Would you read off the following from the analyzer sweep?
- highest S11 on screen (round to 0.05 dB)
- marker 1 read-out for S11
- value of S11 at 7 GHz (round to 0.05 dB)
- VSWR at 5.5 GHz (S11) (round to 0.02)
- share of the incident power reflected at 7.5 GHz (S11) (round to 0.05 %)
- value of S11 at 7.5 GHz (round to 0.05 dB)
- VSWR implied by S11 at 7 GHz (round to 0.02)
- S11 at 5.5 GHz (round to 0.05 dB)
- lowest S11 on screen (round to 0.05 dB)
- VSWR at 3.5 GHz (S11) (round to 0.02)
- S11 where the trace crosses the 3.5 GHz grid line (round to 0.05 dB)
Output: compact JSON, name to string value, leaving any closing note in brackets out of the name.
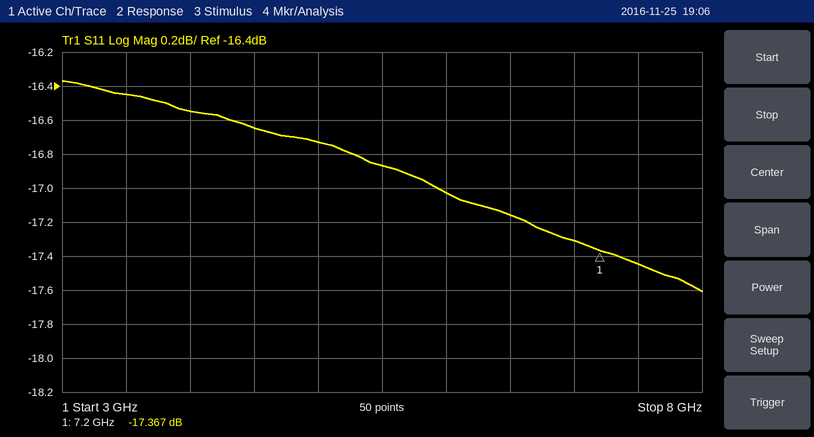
{"highest S11 on screen": "-16.35 dB", "marker 1 read-out for S11": "-17.367 dB", "value of S11 at 7 GHz": "-17.30 dB", "VSWR at 5.5 GHz (S11)": "1.34", "share of the incident power reflected at 7.5 GHz (S11)": "1.80 %", "value of S11 at 7.5 GHz": "-17.45 dB", "VSWR implied by S11 at 7 GHz": "1.32", "S11 at 5.5 GHz": "-16.85 dB", "lowest S11 on screen": "-17.60 dB", "VSWR at 3.5 GHz (S11)": "1.36", "S11 where the trace crosses the 3.5 GHz grid line": "-16.45 dB"}
